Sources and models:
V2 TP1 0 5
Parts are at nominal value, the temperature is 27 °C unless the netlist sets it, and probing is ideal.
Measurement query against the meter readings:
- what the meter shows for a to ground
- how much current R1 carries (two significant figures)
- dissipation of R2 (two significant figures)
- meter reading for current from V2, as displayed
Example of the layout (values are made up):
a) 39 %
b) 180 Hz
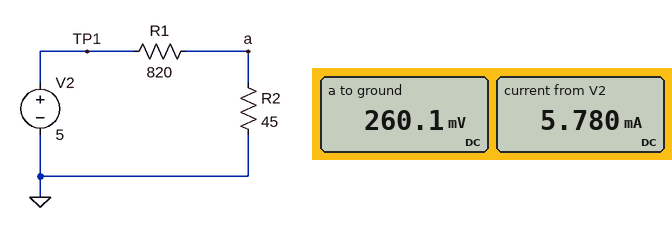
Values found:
a) 260.1 mV
b) 5.8 mA
c) 1.5 mW
d) 5.780 mA
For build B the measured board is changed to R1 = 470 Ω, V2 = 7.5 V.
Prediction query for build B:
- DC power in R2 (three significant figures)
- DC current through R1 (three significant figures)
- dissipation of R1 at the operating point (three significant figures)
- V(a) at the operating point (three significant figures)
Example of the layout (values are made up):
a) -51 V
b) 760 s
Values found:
a) 9.54 mW
b) 14.6 mA
c) 99.7 mW
d) 655 mV
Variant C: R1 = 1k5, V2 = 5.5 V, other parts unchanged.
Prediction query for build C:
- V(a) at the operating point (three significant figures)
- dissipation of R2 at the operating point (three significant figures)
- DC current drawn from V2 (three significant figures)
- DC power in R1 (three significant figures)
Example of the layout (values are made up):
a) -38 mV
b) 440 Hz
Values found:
a) 160 mV
b) 570 µW
c) 3.56 mA
d) 19.0 mW
